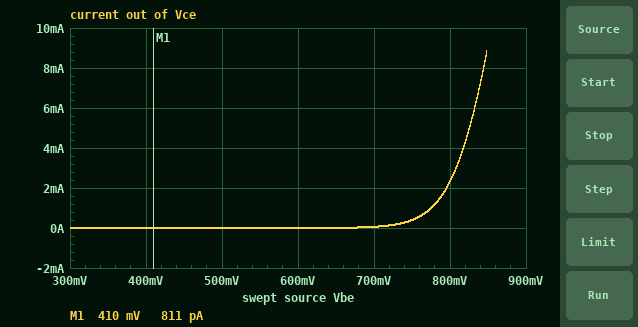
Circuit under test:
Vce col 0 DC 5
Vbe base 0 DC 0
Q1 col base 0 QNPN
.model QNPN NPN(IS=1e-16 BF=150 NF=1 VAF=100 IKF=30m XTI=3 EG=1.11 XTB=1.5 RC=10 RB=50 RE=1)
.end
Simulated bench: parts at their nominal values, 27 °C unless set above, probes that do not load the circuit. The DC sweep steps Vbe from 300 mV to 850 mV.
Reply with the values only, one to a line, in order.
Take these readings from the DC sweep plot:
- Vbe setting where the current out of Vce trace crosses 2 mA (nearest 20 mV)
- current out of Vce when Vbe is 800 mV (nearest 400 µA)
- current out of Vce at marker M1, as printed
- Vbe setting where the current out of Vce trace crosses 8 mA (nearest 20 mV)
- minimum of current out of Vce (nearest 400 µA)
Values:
800 mV
2.4 mA
811 pA
840 mV
0 A
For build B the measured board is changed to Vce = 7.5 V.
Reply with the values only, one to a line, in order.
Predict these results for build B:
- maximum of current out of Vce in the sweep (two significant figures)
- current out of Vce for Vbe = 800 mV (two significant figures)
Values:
9.3 mA
2.4 mA
